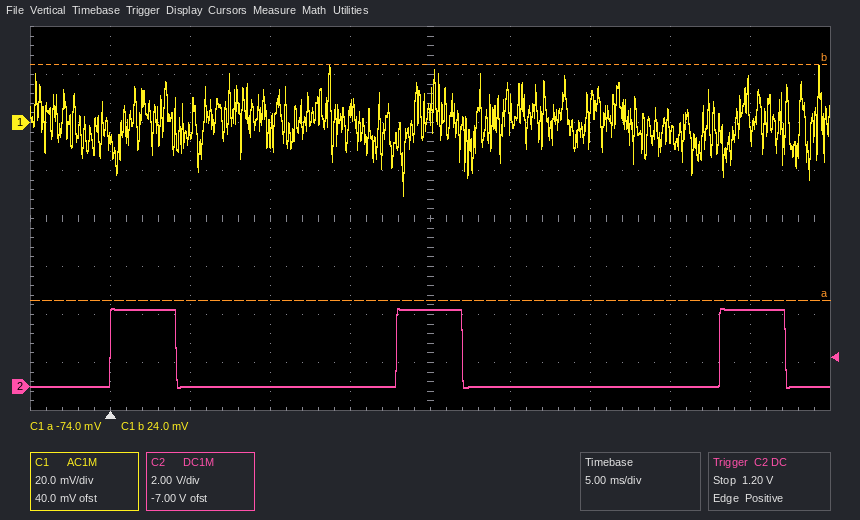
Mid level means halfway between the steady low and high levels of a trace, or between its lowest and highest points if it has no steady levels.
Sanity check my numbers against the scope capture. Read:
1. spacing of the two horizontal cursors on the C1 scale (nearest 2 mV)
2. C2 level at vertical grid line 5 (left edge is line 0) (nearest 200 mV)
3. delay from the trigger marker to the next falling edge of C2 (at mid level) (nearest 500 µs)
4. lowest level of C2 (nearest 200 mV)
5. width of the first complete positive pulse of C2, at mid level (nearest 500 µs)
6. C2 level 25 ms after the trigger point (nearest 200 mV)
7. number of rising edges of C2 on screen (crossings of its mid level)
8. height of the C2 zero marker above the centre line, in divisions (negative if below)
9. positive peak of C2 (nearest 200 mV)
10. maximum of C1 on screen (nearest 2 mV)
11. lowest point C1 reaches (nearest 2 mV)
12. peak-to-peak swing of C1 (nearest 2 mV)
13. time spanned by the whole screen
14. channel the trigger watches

98 mV
3.2 V
4.0 ms
0.0 V
4.0 ms
0.0 V
3
-3.5 div
3.2 V
24 mV
-30 mV
54 mV
50 ms
C2
